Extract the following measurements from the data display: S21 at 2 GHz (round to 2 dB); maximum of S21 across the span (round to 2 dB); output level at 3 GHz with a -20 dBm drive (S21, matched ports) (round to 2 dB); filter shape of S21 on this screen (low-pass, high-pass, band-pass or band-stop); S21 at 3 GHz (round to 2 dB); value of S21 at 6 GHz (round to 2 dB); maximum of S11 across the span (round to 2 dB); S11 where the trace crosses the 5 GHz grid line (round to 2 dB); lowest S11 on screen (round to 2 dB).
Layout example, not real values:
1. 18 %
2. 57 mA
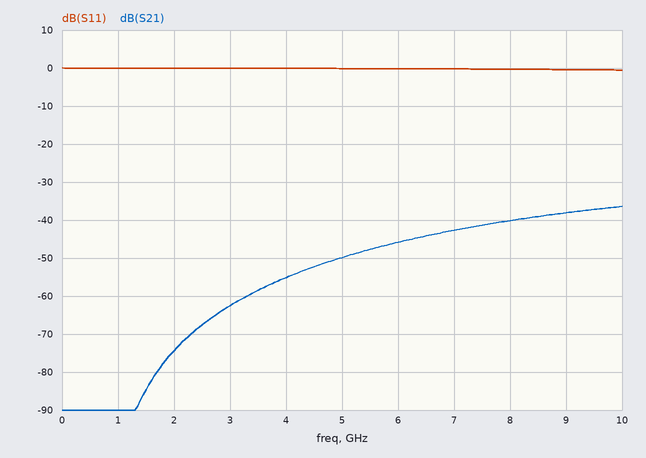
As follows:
1. -74 dB
2. -36 dB
3. -82 dBm
4. high-pass
5. -62 dB
6. -46 dB
7. 0 dB
8. 0 dB
9. 0 dB
